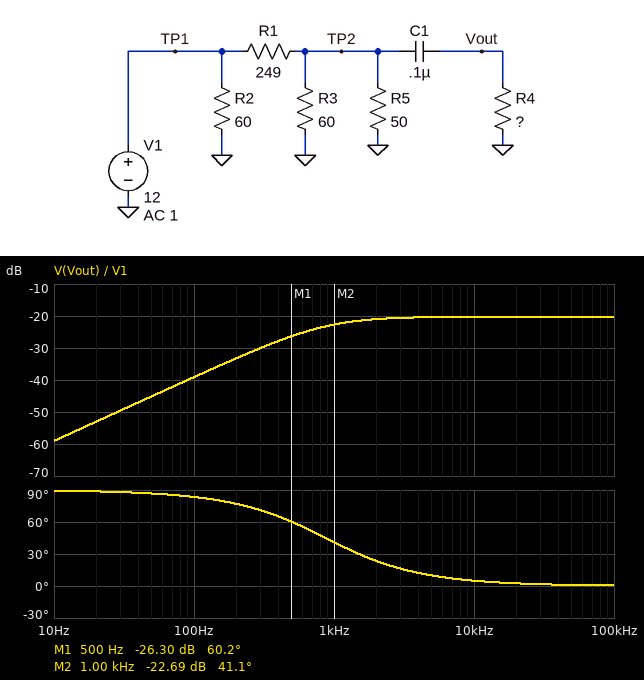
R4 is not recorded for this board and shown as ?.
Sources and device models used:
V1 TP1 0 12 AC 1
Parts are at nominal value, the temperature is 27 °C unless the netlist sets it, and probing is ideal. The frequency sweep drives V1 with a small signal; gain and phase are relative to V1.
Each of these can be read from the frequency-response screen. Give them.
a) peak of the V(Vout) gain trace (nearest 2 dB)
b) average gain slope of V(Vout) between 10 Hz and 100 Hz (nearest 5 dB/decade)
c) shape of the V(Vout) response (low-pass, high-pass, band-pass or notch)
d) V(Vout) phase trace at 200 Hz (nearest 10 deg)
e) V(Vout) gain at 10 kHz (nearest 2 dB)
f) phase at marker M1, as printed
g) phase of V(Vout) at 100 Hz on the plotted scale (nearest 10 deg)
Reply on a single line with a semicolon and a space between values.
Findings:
-20 dB; 20 dB/decade; high-pass; 80 deg; -20 dB; 60.2 deg; 80 deg
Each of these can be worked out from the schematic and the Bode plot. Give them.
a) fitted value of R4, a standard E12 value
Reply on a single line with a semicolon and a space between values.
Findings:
1.8 kΩ
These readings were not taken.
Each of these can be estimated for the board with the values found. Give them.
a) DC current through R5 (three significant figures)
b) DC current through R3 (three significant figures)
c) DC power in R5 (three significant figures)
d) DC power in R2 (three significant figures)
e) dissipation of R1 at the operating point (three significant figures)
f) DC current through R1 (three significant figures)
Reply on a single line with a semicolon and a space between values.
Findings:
23.7 mA; 19.7 mA; 28.1 mW; 2.40 W; 470 mW; 43.4 mA
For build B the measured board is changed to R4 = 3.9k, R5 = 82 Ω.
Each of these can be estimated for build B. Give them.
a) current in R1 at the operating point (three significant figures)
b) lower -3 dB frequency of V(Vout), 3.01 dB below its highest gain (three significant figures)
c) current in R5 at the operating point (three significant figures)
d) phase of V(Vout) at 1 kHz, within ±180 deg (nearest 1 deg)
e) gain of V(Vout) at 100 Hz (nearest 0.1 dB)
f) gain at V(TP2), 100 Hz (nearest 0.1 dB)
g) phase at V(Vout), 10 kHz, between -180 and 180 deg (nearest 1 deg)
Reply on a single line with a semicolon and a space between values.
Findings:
42.3 mA; 405 Hz; 17.9 mA; 22 deg; -30.7 dB; -18.3 dB; 2 deg
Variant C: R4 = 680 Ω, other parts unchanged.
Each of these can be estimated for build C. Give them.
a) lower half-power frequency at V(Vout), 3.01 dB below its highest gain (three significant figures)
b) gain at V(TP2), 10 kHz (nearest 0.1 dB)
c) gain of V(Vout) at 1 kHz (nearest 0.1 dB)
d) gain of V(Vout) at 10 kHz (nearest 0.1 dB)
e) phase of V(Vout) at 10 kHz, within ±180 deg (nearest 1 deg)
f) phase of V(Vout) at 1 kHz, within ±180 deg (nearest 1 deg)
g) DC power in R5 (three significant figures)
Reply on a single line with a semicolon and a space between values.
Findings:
2.26 kHz; -20.4 dB; -28.3 dB; -20.6 dB; 13 deg; 66 deg; 28.1 mW
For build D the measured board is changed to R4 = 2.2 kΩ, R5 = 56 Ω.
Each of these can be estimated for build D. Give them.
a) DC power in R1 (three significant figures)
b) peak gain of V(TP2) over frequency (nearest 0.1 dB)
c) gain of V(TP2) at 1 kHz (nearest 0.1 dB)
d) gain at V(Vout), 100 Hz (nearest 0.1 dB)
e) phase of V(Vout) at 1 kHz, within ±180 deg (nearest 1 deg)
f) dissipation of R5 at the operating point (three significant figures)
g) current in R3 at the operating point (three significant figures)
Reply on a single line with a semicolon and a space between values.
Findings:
464 mW; -19.6 dB; -19.7 dB; -36.9 dB; 36 deg; 27.9 mW; 20.8 mA
